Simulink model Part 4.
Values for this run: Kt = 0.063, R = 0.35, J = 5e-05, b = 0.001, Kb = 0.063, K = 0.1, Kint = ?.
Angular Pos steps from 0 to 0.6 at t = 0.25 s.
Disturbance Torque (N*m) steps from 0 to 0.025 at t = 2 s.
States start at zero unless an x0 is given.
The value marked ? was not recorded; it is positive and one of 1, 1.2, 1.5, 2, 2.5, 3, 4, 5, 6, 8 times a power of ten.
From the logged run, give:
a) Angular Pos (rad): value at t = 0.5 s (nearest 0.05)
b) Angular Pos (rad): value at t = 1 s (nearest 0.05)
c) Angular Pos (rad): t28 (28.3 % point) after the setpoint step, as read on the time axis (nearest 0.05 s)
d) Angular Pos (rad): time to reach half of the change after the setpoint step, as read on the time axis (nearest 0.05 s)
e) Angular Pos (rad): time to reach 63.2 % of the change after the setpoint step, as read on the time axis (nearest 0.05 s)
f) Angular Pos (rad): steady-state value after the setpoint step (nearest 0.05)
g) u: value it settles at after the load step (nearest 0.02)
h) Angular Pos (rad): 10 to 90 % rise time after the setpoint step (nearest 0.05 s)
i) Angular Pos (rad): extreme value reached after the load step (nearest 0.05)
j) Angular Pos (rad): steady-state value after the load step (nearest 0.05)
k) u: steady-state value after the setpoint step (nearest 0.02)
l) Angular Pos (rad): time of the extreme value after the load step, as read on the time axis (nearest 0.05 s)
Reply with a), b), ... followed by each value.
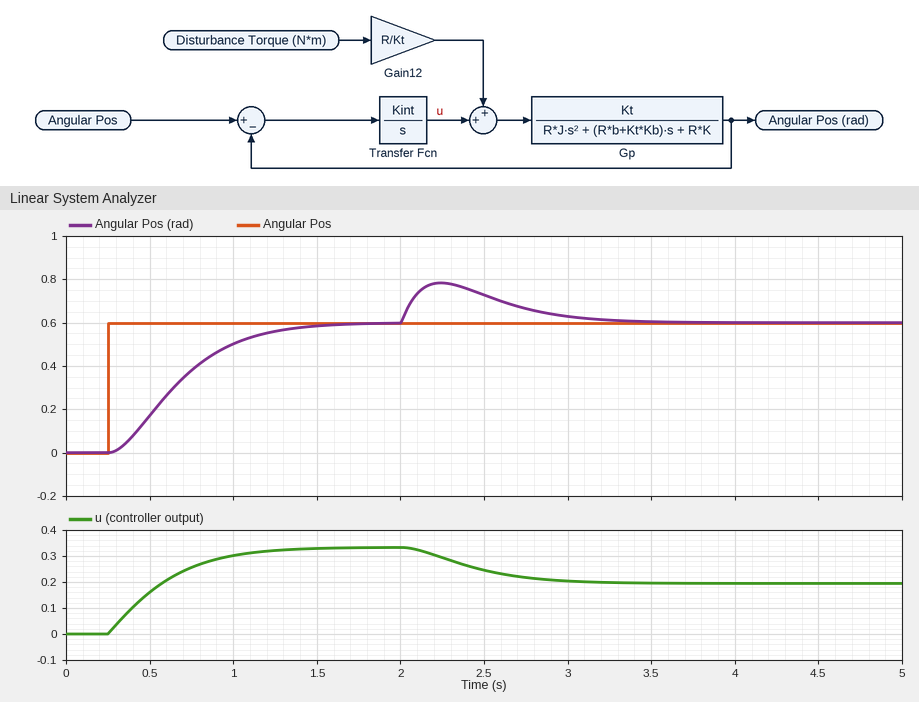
a) 0.15
b) 0.50
c) 0.50 s
d) 0.65 s
e) 0.75 s
f) 0.60
g) 0.20
h) 0.75 s
i) 0.80
j) 0.60
k) 0.34
l) 2.25 s
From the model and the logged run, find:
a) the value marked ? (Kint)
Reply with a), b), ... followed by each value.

a) 1.2
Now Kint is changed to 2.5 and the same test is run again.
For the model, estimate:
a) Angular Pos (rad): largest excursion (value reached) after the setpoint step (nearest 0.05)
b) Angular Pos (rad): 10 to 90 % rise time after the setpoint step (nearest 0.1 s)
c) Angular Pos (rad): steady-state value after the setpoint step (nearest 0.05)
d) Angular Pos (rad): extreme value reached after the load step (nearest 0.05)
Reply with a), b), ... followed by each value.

a) 0.65
b) 0.3 s
c) 0.60
d) 0.75
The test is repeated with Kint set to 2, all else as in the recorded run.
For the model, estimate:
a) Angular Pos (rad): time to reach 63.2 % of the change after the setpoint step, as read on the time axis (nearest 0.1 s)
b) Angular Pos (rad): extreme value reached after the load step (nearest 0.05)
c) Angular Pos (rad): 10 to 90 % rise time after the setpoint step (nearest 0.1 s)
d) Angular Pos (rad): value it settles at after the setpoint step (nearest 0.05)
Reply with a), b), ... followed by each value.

a) 0.6 s
b) 0.75
c) 0.4 s
d) 0.60
